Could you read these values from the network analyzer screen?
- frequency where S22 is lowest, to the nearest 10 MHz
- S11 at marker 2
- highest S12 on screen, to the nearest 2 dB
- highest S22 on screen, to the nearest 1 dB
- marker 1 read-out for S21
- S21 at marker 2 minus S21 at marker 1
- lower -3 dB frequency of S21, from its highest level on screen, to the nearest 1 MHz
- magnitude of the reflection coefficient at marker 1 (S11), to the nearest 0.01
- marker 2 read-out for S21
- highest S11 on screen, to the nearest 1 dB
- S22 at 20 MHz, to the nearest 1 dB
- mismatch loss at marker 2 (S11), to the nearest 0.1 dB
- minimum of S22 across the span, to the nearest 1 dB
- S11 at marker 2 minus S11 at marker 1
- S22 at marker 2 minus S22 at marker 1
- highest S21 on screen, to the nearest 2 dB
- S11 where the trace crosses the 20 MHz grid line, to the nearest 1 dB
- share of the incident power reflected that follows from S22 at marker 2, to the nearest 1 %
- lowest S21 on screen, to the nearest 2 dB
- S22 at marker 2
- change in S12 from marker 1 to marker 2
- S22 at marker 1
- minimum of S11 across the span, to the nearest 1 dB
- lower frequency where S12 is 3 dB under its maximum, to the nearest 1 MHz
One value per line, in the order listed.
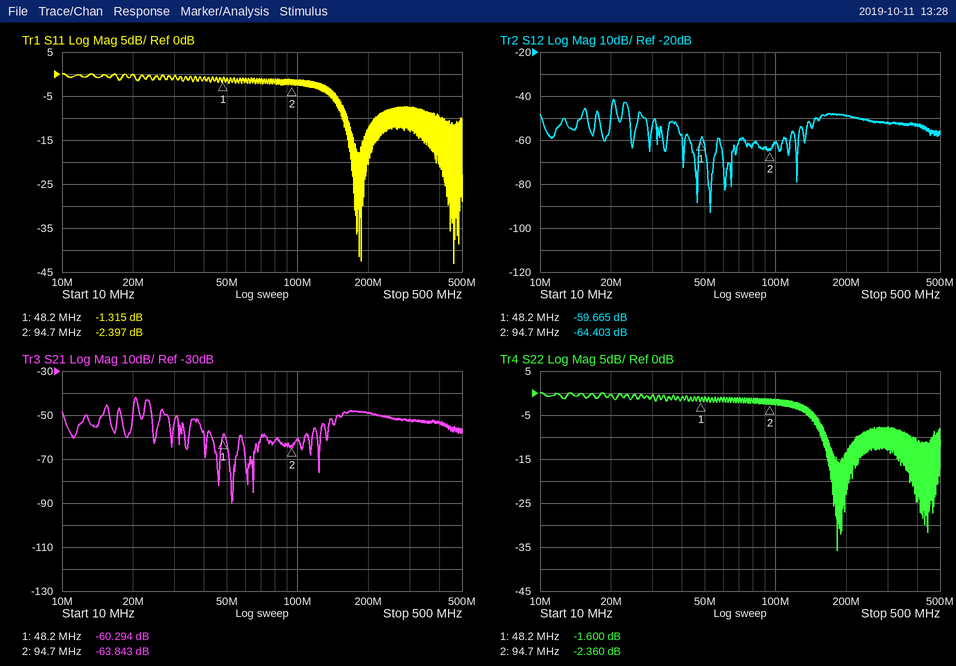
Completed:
180 MHz
-2.397 dB
-42 dB
0 dB
-60.294 dB
-3.549 dB
20 MHz
0.86
-63.843 dB
0 dB
0 dB
3.7 dB
-36 dB
-1.082 dB
-0.760 dB
-42 dB
0 dB
58 %
-90 dB
-2.360 dB
-4.738 dB
-1.600 dB
-43 dB
20 MHz
